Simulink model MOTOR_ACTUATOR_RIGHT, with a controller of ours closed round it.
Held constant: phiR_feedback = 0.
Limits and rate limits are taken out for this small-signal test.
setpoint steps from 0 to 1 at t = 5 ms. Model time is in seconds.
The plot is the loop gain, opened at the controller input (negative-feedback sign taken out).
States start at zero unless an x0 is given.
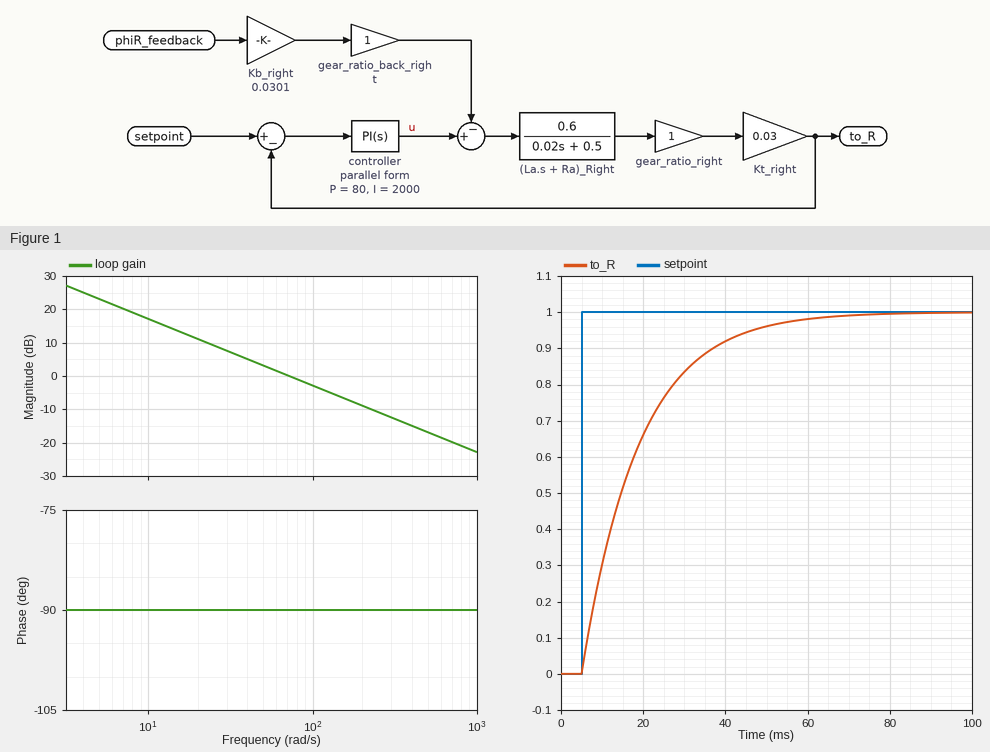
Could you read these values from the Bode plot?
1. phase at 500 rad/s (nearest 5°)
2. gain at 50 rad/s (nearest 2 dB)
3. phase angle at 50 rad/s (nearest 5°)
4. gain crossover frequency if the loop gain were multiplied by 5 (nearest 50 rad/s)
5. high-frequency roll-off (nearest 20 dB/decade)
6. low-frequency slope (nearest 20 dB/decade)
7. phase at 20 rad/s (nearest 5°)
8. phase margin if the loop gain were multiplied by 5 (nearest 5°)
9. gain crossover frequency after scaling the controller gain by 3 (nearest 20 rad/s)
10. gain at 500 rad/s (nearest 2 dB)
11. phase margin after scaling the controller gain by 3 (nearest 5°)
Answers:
-90°
4 dB
-90°
350 rad/s
-20 dB/decade
-20 dB/decade
-90°
90°
220 rad/s
-16 dB
90°
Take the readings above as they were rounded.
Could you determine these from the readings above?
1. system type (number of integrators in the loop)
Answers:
1
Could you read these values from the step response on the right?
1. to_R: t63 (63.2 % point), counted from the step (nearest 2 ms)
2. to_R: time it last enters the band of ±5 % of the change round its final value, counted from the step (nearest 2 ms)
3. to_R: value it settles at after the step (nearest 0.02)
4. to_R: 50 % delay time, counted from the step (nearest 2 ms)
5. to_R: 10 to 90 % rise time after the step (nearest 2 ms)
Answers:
14 ms
42 ms
1.00
10 ms
30 ms
